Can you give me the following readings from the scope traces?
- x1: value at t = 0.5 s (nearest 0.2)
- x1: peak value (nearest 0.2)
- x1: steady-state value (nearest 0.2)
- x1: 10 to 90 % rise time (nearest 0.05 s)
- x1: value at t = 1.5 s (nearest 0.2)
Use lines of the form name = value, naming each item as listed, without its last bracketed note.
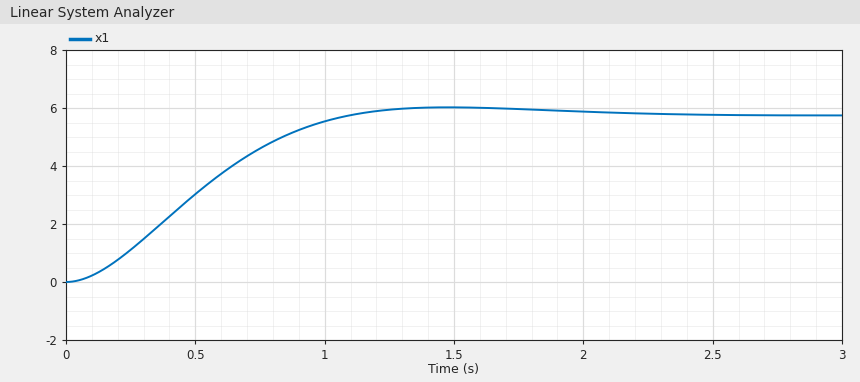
x1: value at t = 0.5 s = 3.0
x1: peak value = 6.0
x1: steady-state value = 5.8
x1: 10 to 90 % rise time = 0.70 s
x1: value at t = 1.5 s = 6.0
